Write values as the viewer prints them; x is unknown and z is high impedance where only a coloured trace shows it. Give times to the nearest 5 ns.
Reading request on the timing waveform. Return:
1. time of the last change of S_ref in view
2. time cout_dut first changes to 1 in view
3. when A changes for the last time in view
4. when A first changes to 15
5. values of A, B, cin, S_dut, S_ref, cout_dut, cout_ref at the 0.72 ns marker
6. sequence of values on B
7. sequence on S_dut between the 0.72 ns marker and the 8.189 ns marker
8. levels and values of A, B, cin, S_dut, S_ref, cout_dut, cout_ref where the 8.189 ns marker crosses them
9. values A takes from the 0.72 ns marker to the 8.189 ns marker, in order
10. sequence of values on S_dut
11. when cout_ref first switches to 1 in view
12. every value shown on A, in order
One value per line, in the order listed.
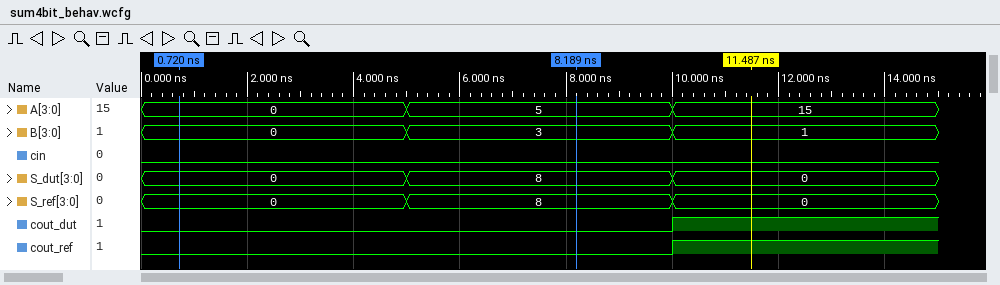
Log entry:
10 ns
10 ns
10 ns
10 ns
A=0, B=0, cin=0, S_dut=0, S_ref=0, cout_dut=0, cout_ref=0
0, 3, 1
0, 8
A=5, B=3, cin=0, S_dut=8, S_ref=8, cout_dut=0, cout_ref=0
0, 5
0, 8, 0
10 ns
0, 5, 15
